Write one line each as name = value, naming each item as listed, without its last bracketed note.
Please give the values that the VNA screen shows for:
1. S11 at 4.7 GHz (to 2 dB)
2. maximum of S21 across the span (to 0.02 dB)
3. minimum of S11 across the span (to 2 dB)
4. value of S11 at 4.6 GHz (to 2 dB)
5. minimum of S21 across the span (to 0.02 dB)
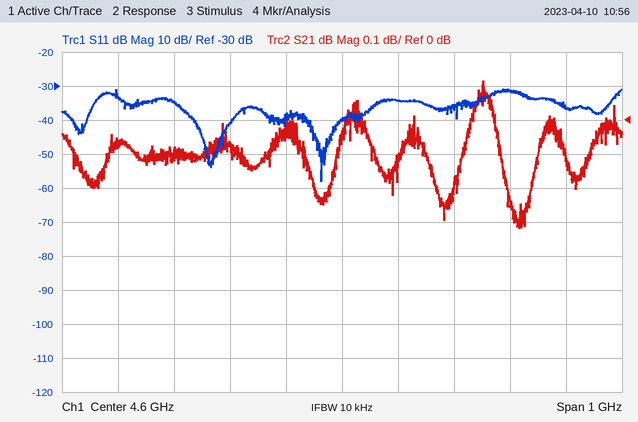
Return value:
S11 at 4.7 GHz = -34 dB
maximum of S21 across the span = 0.12 dB
minimum of S11 across the span = -58 dB
value of S11 at 4.6 GHz = -40 dB
minimum of S21 across the span = -0.32 dB
